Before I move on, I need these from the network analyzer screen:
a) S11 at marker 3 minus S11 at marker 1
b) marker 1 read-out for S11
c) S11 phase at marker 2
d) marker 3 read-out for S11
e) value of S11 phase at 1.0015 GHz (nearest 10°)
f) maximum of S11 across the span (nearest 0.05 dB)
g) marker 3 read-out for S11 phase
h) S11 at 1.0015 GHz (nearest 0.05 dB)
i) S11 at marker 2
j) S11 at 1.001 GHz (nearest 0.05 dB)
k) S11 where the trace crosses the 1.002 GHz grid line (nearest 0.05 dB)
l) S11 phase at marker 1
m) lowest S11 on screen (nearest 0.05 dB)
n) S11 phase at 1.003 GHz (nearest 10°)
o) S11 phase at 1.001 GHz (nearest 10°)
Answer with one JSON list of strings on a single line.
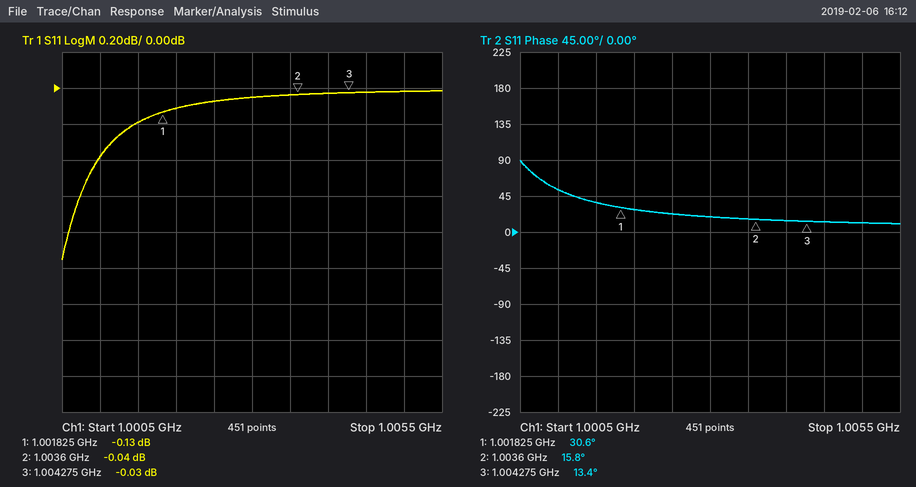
["0.10 dB", "-0.13 dB", "15.8°", "-0.03 dB", "40°", "0.00 dB", "13.4°", "-0.20 dB", "-0.04 dB", "-0.40 dB", "-0.10 dB", "30.6°", "-0.95 dB", "20°", "50°"]
